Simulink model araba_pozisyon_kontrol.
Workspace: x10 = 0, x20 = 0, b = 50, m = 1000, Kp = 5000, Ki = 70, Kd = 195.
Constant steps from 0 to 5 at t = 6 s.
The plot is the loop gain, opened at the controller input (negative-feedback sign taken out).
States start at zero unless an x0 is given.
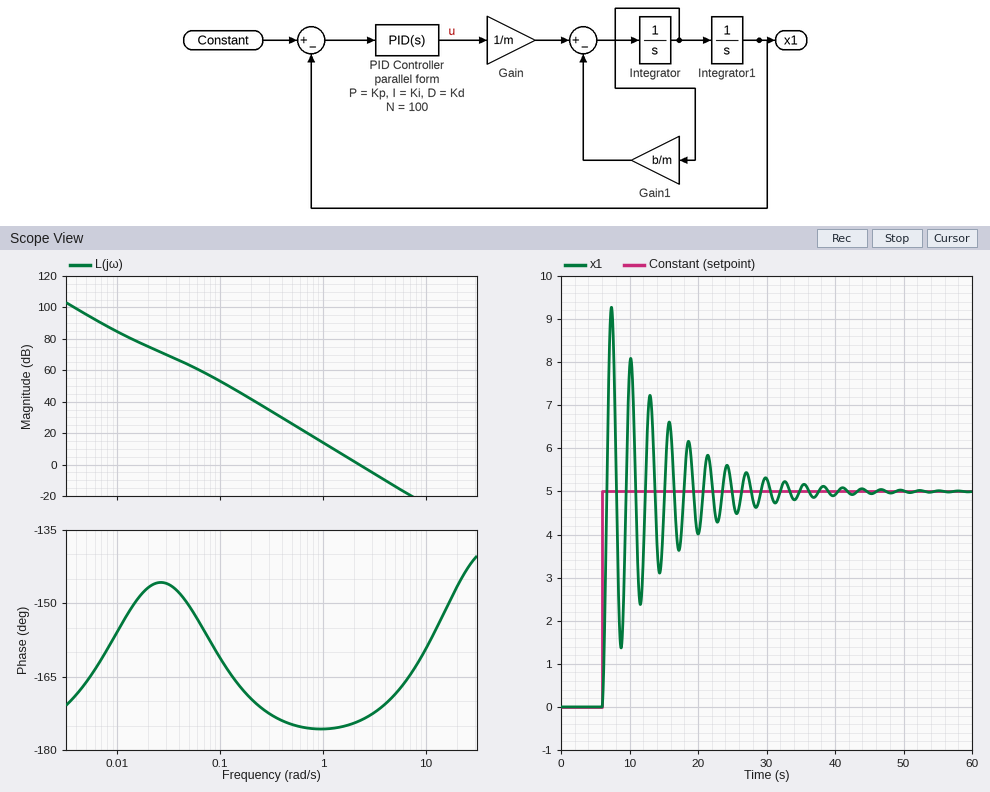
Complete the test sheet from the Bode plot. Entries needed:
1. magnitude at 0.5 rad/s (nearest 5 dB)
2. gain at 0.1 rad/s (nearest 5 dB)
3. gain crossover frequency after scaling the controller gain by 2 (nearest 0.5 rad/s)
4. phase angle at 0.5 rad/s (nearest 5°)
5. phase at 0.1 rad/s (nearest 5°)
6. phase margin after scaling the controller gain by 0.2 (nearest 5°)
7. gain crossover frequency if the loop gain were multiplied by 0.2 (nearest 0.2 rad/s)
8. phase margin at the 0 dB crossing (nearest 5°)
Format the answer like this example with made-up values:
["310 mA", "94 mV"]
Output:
["25 dB", "55 dB", "3.0 rad/s", "-175°", "-160°", "5°", "1.0 rad/s", "5°"]
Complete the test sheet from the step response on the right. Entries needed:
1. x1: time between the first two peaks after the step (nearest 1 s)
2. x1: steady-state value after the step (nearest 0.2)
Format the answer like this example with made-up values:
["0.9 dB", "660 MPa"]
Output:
["3 s", "5.0"]
